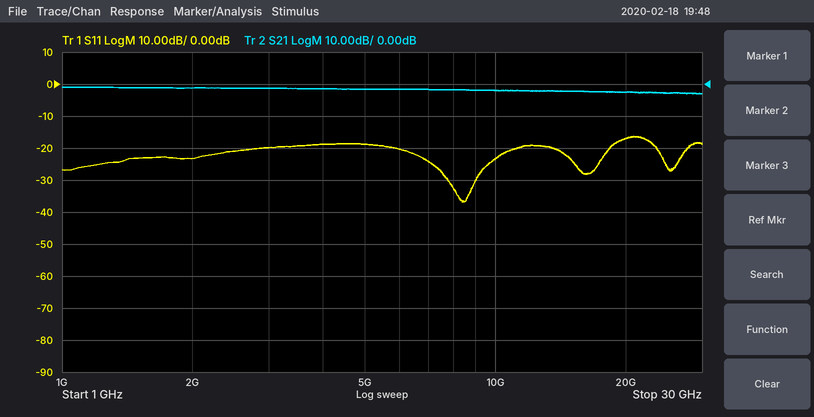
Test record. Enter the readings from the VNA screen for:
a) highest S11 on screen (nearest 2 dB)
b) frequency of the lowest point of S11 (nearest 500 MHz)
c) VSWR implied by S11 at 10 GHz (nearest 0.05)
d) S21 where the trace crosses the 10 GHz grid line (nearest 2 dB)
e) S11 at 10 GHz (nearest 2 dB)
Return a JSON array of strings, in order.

["-16 dB", "8.5 GHz", "1.15", "-2 dB", "-24 dB"]
